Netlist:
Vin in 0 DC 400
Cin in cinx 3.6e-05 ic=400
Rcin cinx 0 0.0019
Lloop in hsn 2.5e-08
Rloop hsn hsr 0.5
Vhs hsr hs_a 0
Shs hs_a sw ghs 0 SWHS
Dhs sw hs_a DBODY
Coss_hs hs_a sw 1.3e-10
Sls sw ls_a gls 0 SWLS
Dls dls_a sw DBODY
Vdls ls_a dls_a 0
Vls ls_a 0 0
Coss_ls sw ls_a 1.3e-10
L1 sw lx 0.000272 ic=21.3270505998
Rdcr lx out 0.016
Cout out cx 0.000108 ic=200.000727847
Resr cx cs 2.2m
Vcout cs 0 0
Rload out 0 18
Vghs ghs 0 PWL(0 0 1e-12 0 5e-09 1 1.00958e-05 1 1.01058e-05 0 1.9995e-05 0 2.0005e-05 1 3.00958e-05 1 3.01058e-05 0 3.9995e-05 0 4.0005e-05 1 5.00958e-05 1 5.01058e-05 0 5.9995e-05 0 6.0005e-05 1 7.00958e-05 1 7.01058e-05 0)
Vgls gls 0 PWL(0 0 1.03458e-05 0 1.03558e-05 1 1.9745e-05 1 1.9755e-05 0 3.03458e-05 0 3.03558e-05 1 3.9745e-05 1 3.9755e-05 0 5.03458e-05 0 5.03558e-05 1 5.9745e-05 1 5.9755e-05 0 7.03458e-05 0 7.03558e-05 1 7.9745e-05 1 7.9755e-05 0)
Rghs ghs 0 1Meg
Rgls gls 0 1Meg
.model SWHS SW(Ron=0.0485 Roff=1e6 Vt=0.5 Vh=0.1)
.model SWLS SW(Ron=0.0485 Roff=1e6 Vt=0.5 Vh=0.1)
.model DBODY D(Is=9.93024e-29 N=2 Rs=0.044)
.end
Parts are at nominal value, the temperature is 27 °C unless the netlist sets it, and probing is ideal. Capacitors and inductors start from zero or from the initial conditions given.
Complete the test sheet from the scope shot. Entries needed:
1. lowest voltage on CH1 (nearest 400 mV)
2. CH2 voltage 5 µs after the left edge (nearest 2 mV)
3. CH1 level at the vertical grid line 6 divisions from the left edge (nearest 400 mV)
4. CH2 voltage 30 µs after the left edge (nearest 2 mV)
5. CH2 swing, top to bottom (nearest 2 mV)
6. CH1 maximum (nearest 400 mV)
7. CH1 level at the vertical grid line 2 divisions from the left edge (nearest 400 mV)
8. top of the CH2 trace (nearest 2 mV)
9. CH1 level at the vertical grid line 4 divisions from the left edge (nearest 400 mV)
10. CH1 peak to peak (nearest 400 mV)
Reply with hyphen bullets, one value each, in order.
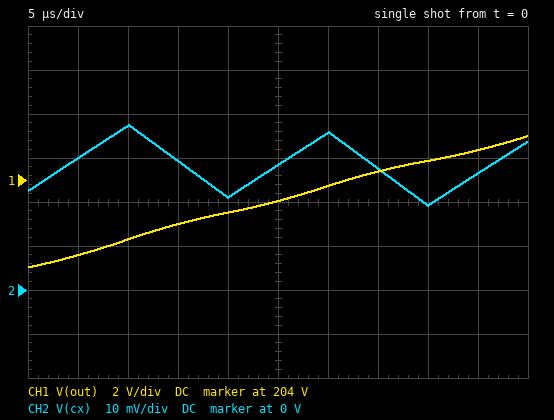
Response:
- 200.0 V
- 30 mV
- 203.6 V
- 36 mV
- 18 mV
- 206.0 V
- 201.2 V
- 38 mV
- 202.4 V
- 6.0 V
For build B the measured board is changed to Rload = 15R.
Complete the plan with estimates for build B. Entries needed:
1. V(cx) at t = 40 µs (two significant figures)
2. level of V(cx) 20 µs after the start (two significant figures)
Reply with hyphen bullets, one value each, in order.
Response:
- 14 mV
- 16 mV
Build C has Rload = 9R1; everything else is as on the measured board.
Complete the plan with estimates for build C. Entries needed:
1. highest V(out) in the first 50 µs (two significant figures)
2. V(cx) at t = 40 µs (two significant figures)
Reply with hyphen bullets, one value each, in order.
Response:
- 200 V
- -3.7 mV
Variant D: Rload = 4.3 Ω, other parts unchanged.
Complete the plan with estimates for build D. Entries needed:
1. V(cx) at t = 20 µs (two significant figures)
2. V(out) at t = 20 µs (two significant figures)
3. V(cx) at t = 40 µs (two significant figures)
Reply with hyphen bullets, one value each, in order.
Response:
- -54 mV
- 200 V
- -52 mV
